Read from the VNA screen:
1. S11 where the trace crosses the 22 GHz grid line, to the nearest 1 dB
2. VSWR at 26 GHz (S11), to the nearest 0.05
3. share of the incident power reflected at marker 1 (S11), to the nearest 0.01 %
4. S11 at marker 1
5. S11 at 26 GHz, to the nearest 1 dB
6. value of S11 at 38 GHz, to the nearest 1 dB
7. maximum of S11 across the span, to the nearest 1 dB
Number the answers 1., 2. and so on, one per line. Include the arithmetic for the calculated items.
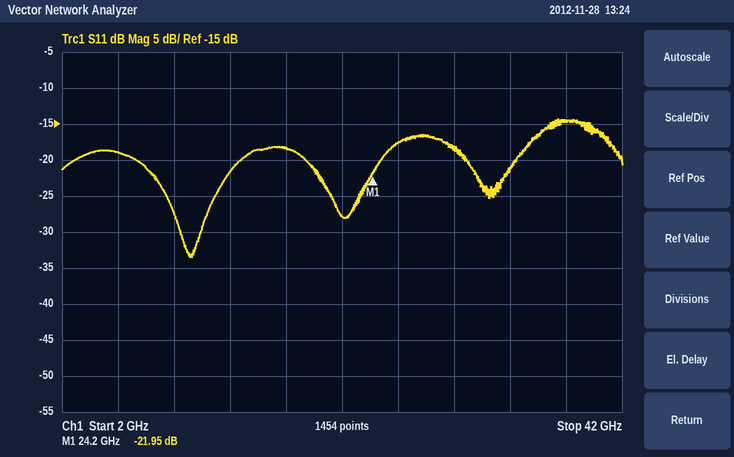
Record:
1. -28 dB
2. |Γ| = 10^(-18/20) = 0.1259; VSWR = (1 + 0.1259)/(1 − 0.1259) ≈ 1.29, so 1.30 to the nearest 0.05
3. 10^(-21.95/10) ≈ 0.64 %
4. -21.95 dB
5. -18 dB
6. -15 dB
7. -14 dB
